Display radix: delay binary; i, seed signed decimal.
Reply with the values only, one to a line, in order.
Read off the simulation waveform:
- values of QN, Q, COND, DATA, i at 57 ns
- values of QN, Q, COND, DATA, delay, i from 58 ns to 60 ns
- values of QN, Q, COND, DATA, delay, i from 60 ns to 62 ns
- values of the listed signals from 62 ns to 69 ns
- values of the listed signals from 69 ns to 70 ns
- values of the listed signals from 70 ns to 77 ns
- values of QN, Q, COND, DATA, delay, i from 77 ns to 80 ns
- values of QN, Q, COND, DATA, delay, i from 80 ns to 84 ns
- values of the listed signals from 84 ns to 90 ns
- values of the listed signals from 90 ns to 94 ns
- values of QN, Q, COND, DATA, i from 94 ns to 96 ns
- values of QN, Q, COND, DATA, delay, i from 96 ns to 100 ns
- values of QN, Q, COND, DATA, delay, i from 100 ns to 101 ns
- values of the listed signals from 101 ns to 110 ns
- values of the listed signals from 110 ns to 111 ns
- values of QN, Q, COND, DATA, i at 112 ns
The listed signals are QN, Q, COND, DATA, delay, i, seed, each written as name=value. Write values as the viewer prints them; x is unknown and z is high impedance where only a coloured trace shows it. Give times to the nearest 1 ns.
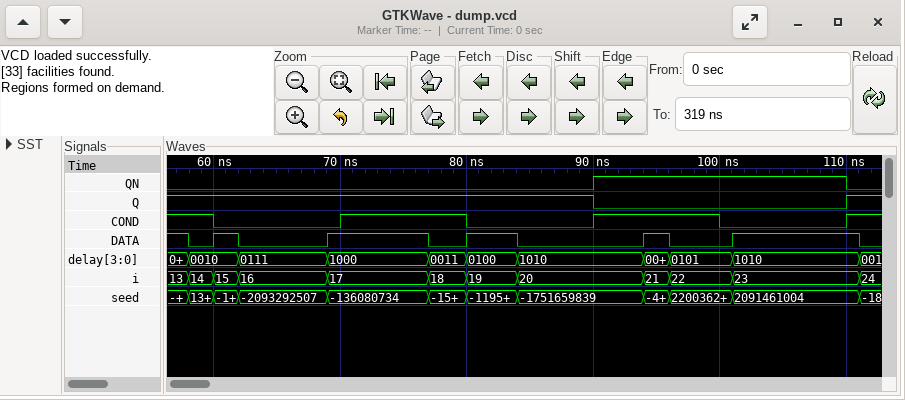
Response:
QN=0, Q=1, COND=1, DATA=1, i=13
QN=0, Q=1, COND=1, DATA=0, delay=0010, i=14
QN=0, Q=1, COND=0, DATA=1, delay=0010, i=15
QN=0, Q=1, COND=0, DATA=0, delay=0111, i=16, seed=-2093292507
QN=0, Q=1, COND=0, DATA=1, delay=1000, i=17, seed=-136080734
QN=0, Q=1, COND=1, DATA=1, delay=1000, i=17, seed=-136080734
QN=0, Q=1, COND=1, DATA=0, delay=0011, i=18
QN=0, Q=1, COND=0, DATA=1, delay=0100, i=19
QN=0, Q=1, COND=0, DATA=0, delay=1010, i=20, seed=-1751659839
QN=1, Q=0, COND=1, DATA=0, delay=1010, i=20, seed=-1751659839
QN=1, Q=0, COND=1, DATA=1, i=21
QN=1, Q=0, COND=1, DATA=0, delay=0101, i=22
QN=1, Q=0, COND=0, DATA=0, delay=0101, i=22
QN=1, Q=0, COND=0, DATA=1, delay=1010, i=23, seed=2091461004
QN=0, Q=1, COND=1, DATA=1, delay=1010, i=23, seed=2091461004
QN=0, Q=1, COND=1, DATA=0, i=24
